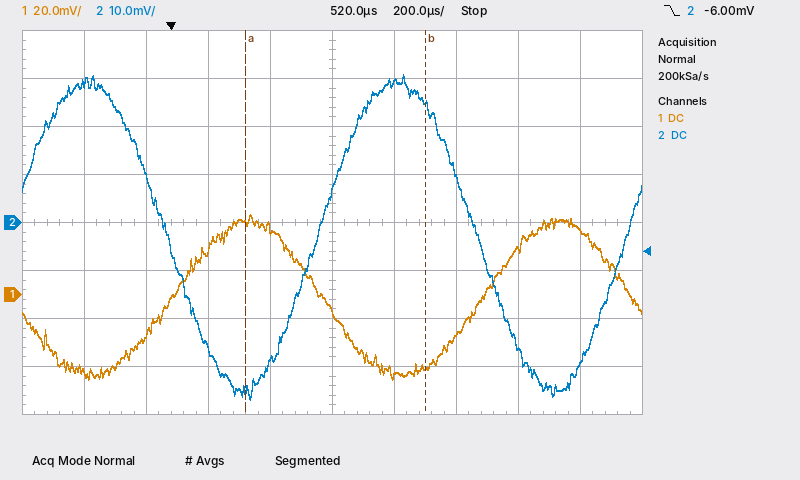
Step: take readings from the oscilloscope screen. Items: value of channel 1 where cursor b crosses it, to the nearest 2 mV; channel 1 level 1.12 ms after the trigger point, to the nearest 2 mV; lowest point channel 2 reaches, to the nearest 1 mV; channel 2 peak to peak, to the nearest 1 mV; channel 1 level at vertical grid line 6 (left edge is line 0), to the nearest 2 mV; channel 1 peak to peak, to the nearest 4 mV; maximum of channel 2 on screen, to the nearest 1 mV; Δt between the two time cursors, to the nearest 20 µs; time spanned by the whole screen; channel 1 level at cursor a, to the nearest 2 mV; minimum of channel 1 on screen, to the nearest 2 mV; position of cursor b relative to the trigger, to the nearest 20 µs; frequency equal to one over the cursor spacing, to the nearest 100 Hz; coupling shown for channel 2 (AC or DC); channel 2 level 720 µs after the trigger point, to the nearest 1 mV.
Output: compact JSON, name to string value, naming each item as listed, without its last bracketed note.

{"value of channel 1 where cursor b crosses it, to the nearest 2 mV": "-30 mV", "channel 1 level 1.12 ms after the trigger point, to the nearest 2 mV": "20 mV", "lowest point channel 2 reaches, to the nearest 1 mV": "-37 mV", "channel 2 peak to peak, to the nearest 1 mV": "68 mV", "channel 1 level at vertical grid line 6 (left edge is line 0), to the nearest 2 mV": "-34 mV", "channel 1 peak to peak, to the nearest 4 mV": "68 mV", "maximum of channel 2 on screen, to the nearest 1 mV": "31 mV", "Δt between the two time cursors, to the nearest 20 µs": "580 µs", "time spanned by the whole screen": "2 ms", "channel 1 level at cursor a, to the nearest 2 mV": "30 mV", "minimum of channel 1 on screen, to the nearest 2 mV": "-36 mV", "position of cursor b relative to the trigger, to the nearest 20 µs": "+820 µs", "frequency equal to one over the cursor spacing, to the nearest 100 Hz": "1.7 kHz", "coupling shown for channel 2": "DC", "channel 2 level 720 µs after the trigger point, to the nearest 1 mV": "29 mV"}
